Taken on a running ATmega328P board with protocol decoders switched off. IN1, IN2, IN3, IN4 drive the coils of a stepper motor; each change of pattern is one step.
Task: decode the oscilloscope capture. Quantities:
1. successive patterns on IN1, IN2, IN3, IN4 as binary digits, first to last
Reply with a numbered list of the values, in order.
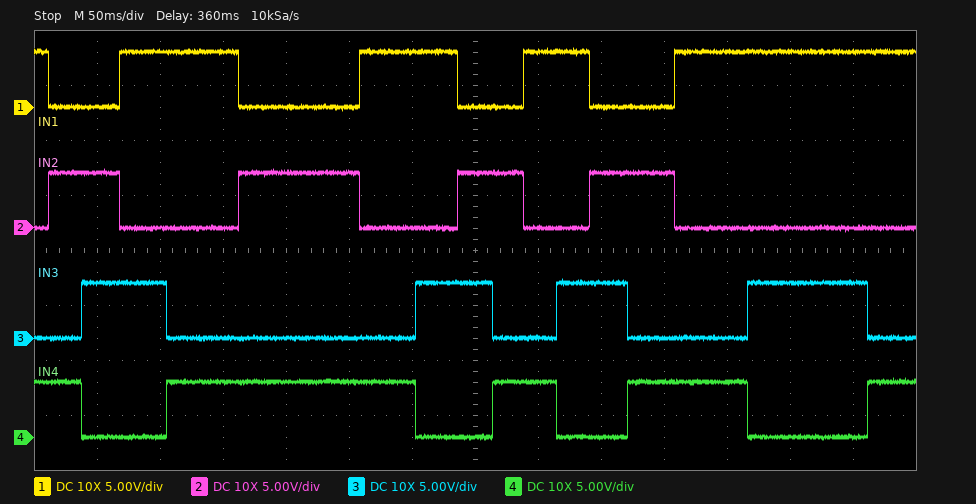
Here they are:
1. 1001 0101 0110 1010 1001 0101 1001 1010 0110 0101 1001 1010 0110 0101 1001 1010 1001
